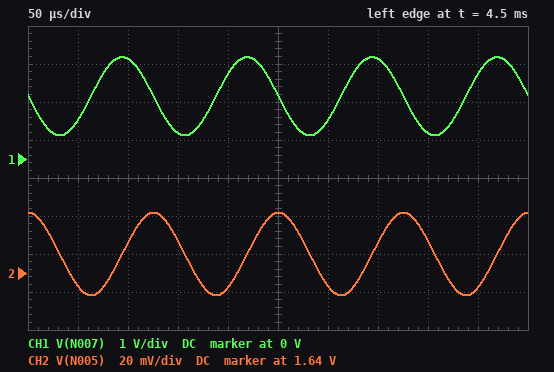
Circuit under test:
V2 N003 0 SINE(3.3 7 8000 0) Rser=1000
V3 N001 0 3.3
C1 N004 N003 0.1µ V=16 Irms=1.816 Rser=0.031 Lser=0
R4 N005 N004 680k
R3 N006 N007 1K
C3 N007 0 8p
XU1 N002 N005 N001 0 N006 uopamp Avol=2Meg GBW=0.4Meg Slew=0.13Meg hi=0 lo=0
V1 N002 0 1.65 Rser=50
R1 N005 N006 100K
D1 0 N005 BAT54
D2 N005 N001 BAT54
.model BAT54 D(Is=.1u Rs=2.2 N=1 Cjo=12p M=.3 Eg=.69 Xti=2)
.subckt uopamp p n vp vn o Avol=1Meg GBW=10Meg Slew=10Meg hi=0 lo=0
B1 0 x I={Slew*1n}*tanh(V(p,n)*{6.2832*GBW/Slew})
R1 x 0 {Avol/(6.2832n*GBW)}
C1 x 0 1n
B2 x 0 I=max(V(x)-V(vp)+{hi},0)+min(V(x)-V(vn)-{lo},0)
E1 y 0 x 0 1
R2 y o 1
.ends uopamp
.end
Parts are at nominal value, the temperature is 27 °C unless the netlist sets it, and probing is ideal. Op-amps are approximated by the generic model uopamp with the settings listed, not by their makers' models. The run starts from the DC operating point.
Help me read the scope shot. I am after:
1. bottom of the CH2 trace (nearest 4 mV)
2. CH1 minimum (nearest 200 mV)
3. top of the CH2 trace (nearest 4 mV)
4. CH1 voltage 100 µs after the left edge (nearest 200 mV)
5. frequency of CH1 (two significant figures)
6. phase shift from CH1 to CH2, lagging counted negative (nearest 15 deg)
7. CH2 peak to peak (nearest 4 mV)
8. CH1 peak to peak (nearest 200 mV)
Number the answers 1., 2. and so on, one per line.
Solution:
1. 1.628 V
2. 600 mV
3. 1.672 V
4. 2.6 V
5. 8.0 kHz
6. -90 deg
7. 44 mV
8. 2.0 V
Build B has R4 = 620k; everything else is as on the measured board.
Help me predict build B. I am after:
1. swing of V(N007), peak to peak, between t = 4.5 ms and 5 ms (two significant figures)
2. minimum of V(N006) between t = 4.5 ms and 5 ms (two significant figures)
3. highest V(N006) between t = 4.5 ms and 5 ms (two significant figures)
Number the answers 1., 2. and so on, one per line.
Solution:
1. 2.3 V
2. 520 mV
3. 2.8 V
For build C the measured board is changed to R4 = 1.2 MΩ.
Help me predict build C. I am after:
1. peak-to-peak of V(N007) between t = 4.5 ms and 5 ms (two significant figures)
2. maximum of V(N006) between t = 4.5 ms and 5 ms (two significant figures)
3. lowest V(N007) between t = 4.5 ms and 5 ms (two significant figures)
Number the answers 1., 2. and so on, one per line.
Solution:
1. 1.2 V
2. 2.2 V
3. 1.1 V
